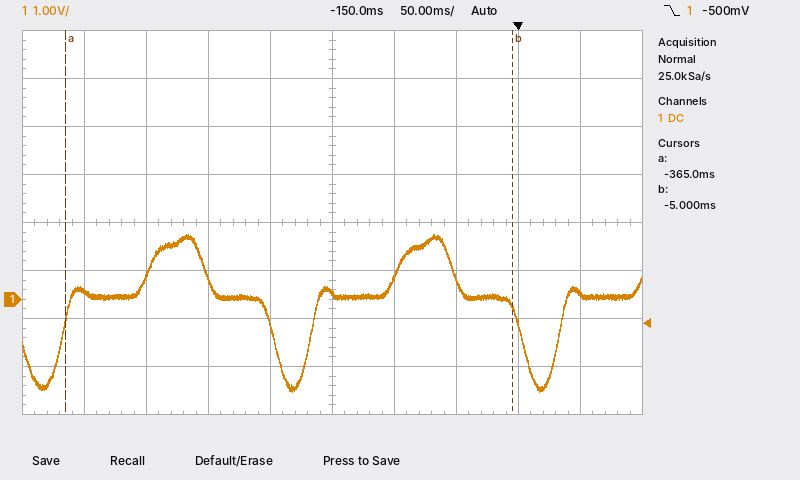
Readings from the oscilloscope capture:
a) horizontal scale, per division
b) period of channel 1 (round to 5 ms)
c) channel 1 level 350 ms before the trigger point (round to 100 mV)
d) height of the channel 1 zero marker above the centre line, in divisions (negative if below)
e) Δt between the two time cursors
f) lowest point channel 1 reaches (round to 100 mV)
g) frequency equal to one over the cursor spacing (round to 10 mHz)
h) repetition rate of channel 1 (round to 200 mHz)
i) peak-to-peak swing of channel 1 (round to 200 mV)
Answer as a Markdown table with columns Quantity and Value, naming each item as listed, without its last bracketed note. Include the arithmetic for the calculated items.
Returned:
| Quantity | Value |
|---|---|
| horizontal scale, per division | 50 ms |
| period of channel 1 | 200 ms |
| channel 1 level 350 ms before the trigger point | 200 mV |
| height of the channel 1 zero marker above the centre line, in divisions | -1.6 div |
| Δt between the two time cursors | -5 ms − (-365 ms) = 360 ms |
| lowest point channel 1 reaches | -1.9 V |
| frequency equal to one over the cursor spacing | 1 / 360 ms ≈ 2.78 Hz |
| repetition rate of channel 1 | 1 / 200 ms ≈ 5.0 Hz |
| peak-to-peak swing of channel 1 | 3.2 V |
